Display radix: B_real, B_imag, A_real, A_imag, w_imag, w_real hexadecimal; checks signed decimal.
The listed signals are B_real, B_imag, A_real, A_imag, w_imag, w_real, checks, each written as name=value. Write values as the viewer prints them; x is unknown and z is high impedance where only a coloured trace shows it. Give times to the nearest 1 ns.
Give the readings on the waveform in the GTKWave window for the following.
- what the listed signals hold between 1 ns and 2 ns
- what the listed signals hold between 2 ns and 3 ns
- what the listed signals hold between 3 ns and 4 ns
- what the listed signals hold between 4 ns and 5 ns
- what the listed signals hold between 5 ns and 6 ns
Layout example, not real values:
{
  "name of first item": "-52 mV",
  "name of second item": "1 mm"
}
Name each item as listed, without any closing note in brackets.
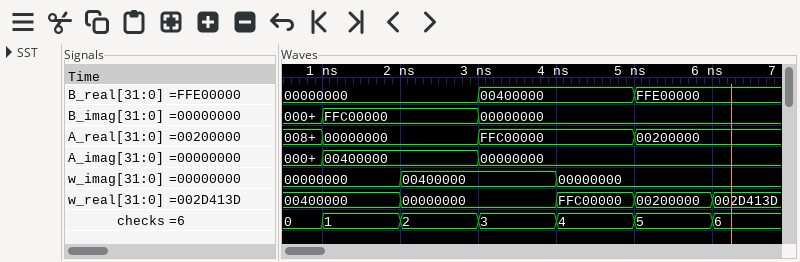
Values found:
{
  "what the listed signals hold between 1 ns and 2 ns": "B_real=00000000, B_imag=FFC00000, A_real=00000000, A_imag=00400000, w_imag=00000000, w_real=00400000, checks=1",
  "what the listed signals hold between 2 ns and 3 ns": "B_real=00000000, B_imag=FFC00000, A_real=00000000, A_imag=00400000, w_imag=00400000, w_real=00000000, checks=2",
  "what the listed signals hold between 3 ns and 4 ns": "B_real=00400000, B_imag=00000000, A_real=FFC00000, A_imag=00000000, w_imag=00400000, w_real=00000000, checks=3",
  "what the listed signals hold between 4 ns and 5 ns": "B_real=00400000, B_imag=00000000, A_real=FFC00000, A_imag=00000000, w_imag=00000000, w_real=FFC00000, checks=4",
  "what the listed signals hold between 5 ns and 6 ns": "B_real=FFE00000, B_imag=00000000, A_real=00200000, A_imag=00000000, w_imag=00000000, w_real=00200000, checks=5"
}
